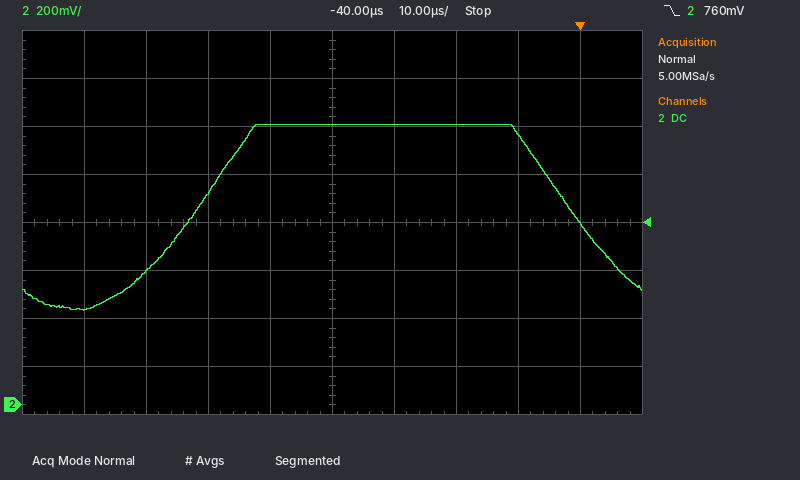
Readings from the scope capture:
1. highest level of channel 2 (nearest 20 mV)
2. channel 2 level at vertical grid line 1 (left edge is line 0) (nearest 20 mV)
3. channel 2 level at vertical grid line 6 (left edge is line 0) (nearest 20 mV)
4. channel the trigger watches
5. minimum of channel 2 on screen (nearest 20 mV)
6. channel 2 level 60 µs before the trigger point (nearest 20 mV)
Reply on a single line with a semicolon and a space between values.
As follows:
1.16 V; 400 mV; 1.16 V; channel 2; 400 mV; 880 mV
